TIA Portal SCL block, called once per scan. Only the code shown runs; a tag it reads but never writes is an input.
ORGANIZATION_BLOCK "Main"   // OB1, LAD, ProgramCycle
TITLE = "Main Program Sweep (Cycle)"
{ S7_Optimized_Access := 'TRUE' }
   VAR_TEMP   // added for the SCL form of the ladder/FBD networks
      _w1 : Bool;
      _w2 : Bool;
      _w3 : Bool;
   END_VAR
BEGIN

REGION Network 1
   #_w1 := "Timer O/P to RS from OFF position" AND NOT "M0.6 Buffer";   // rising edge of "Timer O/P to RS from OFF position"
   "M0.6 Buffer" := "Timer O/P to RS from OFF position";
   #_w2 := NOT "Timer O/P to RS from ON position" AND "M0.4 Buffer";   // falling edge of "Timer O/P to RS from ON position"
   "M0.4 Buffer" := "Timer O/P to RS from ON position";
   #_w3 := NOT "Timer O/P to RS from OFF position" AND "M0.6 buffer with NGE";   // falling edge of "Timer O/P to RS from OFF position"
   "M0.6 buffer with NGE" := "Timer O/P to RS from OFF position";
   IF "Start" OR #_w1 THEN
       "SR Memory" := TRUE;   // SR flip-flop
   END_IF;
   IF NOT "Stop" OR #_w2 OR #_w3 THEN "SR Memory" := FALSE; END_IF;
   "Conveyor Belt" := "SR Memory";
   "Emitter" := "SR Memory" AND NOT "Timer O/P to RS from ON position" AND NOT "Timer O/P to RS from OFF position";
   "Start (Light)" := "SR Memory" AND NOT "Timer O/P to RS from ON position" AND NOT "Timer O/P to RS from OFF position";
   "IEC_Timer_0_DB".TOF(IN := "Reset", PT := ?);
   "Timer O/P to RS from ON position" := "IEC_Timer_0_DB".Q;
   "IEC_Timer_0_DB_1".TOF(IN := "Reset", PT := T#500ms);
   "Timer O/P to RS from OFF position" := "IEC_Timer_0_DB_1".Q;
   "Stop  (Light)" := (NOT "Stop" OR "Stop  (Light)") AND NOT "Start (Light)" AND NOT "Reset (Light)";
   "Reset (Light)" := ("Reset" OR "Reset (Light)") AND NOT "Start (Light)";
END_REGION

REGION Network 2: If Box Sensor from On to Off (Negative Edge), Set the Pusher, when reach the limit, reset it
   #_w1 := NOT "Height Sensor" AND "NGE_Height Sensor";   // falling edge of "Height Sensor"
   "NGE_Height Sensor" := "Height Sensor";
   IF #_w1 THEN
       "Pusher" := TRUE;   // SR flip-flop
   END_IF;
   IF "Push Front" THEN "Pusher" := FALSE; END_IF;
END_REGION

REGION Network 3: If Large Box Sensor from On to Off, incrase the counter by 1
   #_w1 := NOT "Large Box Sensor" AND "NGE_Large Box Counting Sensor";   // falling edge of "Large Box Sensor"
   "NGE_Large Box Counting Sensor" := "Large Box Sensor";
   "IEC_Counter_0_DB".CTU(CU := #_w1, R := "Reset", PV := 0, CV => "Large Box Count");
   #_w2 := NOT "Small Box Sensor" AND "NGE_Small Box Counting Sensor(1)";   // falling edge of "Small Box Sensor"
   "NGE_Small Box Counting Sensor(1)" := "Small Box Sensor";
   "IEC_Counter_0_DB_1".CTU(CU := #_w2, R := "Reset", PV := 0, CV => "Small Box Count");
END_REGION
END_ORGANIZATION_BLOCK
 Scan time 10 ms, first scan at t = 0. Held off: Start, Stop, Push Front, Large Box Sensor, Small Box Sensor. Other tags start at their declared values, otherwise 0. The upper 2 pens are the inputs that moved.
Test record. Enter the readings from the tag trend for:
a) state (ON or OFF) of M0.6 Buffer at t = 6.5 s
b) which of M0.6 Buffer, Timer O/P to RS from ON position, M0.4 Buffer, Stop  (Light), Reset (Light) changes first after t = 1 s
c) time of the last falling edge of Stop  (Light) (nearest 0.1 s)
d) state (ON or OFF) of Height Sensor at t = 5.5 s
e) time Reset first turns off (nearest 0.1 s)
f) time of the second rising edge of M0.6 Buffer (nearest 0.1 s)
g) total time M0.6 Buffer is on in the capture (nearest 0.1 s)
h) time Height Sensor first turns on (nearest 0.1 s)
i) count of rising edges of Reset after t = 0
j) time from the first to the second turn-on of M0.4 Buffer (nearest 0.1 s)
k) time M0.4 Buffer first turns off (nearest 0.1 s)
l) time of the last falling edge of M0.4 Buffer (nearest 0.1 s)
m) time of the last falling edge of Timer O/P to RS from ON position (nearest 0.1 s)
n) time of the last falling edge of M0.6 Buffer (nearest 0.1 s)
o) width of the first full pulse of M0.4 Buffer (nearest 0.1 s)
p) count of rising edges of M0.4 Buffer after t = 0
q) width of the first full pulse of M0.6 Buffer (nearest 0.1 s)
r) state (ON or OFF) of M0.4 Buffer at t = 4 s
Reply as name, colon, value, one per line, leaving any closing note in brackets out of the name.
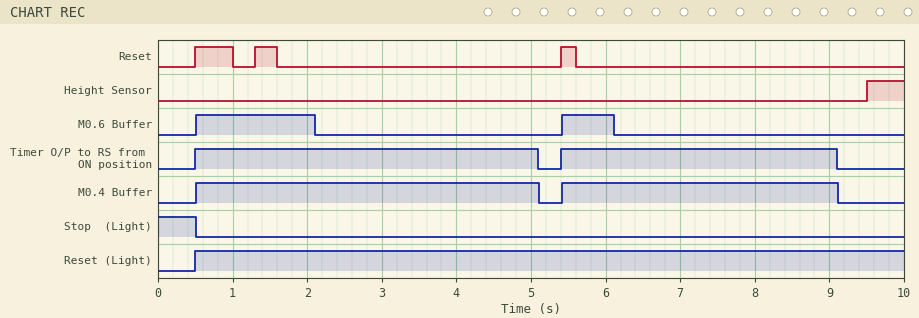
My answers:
state (ON or OFF) of M0.6 Buffer at t = 6.5 s: OFF
which of M0.6 Buffer, Timer O/P to RS from ON position, M0.4 Buffer, Stop  (Light), Reset (Light) changes first after t = 1 s: M0.6 Buffer
time of the last falling edge of Stop  (Light): 0.5 s
state (ON or OFF) of Height Sensor at t = 5.5 s: OFF
time Reset first turns off: 1.0 s
time of the second rising edge of M0.6 Buffer: 5.4 s
total time M0.6 Buffer is on in the capture: 2.3 s
time Height Sensor first turns on: 9.5 s
count of rising edges of Reset after t = 0: 3
time from the first to the second turn-on of M0.4 Buffer: 4.9 s
time M0.4 Buffer first turns off: 5.1 s
time of the last falling edge of M0.4 Buffer: 9.1 s
time of the last falling edge of Timer O/P to RS from ON position: 9.1 s
time of the last falling edge of M0.6 Buffer: 6.1 s
width of the first full pulse of M0.4 Buffer: 4.6 s
count of rising edges of M0.4 Buffer after t = 0: 2
width of the first full pulse of M0.6 Buffer: 1.6 s
state (ON or OFF) of M0.4 Buffer at t = 4 s: ON
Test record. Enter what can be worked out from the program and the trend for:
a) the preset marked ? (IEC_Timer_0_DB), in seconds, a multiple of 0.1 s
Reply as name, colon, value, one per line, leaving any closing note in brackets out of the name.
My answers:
the preset marked ? (IEC_Timer_0_DB), in seconds, a multiple of 0.1 s: 3.5 s
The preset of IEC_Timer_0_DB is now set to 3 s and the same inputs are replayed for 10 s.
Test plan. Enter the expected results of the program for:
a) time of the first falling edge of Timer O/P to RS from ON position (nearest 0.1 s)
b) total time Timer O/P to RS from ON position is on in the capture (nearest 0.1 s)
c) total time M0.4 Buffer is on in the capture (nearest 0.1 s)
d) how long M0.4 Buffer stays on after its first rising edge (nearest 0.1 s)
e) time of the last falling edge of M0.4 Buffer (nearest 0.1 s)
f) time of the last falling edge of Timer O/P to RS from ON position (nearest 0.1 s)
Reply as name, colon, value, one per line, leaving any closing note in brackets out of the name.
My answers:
time of the first falling edge of Timer O/P to RS from ON position: 4.6 s
total time Timer O/P to RS from ON position is on in the capture: 7.3 s
total time M0.4 Buffer is on in the capture: 7.3 s
how long M0.4 Buffer stays on after its first rising edge: 4.1 s
time of the last falling edge of M0.4 Buffer: 8.6 s
time of the last falling edge of Timer O/P to RS from ON position: 8.6 s
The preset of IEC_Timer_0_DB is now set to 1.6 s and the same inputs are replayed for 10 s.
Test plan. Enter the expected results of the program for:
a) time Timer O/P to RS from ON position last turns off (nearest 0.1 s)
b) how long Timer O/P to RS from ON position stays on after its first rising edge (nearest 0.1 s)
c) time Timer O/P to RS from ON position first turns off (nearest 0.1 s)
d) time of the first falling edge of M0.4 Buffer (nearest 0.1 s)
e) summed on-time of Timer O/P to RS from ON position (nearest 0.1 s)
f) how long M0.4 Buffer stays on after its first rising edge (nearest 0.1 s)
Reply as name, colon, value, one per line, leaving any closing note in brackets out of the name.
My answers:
time Timer O/P to RS from ON position last turns off: 7.2 s
how long Timer O/P to RS from ON position stays on after its first rising edge: 2.7 s
time Timer O/P to RS from ON position first turns off: 3.2 s
time of the first falling edge of M0.4 Buffer: 3.2 s
summed on-time of Timer O/P to RS from ON position: 4.5 s
how long M0.4 Buffer stays on after its first rising edge: 2.7 s
